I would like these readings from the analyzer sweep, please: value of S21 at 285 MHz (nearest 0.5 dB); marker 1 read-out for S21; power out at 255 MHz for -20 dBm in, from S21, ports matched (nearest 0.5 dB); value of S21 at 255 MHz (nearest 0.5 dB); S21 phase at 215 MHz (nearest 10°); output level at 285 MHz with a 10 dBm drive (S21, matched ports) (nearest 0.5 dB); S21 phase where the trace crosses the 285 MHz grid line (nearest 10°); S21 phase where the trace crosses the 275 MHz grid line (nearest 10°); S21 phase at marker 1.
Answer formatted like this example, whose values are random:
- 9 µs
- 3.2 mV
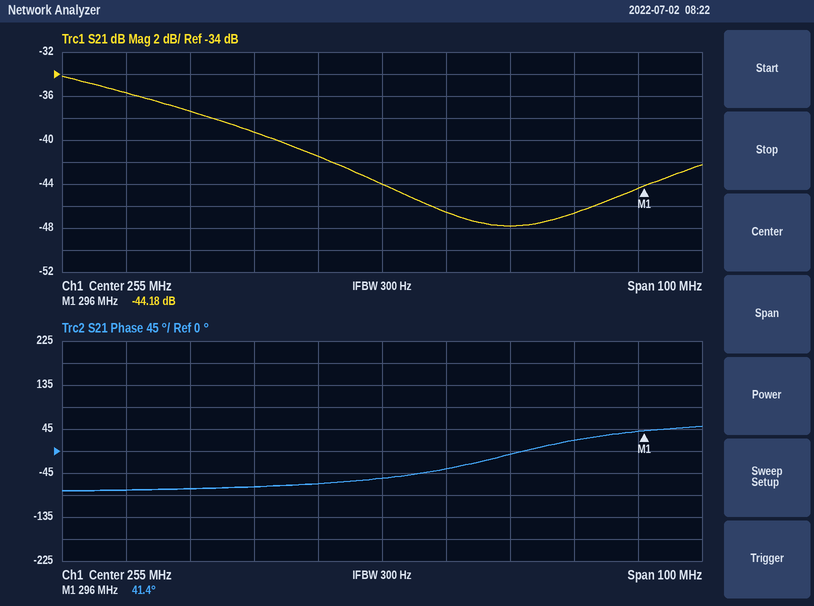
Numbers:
- -46.5 dB
- -44.18 dB
- -64.0 dBm
- -44.0 dB
- -80°
- -36.5 dBm
- 20°
- -10°
- 41.4°
